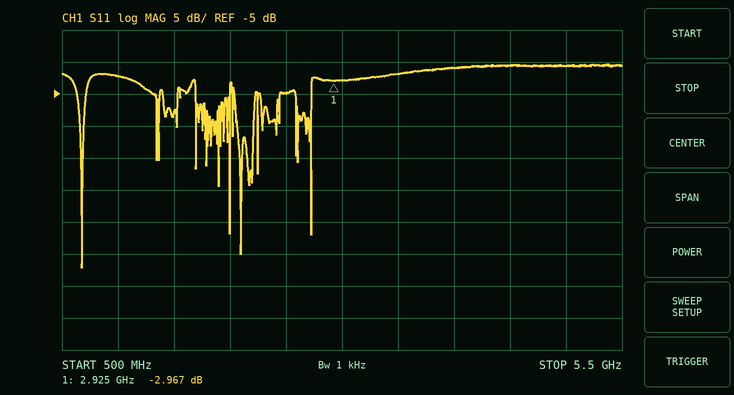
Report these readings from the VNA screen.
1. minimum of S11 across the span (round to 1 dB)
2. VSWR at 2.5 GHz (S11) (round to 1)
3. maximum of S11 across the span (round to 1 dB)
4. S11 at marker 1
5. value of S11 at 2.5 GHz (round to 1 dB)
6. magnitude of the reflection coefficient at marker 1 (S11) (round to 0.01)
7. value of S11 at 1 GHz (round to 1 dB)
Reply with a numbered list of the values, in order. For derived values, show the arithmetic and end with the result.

1. -32 dB
2. |Γ| = 10^(-5/20) = 0.5623; VSWR = (1 + 0.5623)/(1 − 0.5623) ≈ 4
3. 0 dB
4. -2.967 dB
5. -5 dB
6. 10^(-2.967/20) ≈ 0.71
7. -2 dB
